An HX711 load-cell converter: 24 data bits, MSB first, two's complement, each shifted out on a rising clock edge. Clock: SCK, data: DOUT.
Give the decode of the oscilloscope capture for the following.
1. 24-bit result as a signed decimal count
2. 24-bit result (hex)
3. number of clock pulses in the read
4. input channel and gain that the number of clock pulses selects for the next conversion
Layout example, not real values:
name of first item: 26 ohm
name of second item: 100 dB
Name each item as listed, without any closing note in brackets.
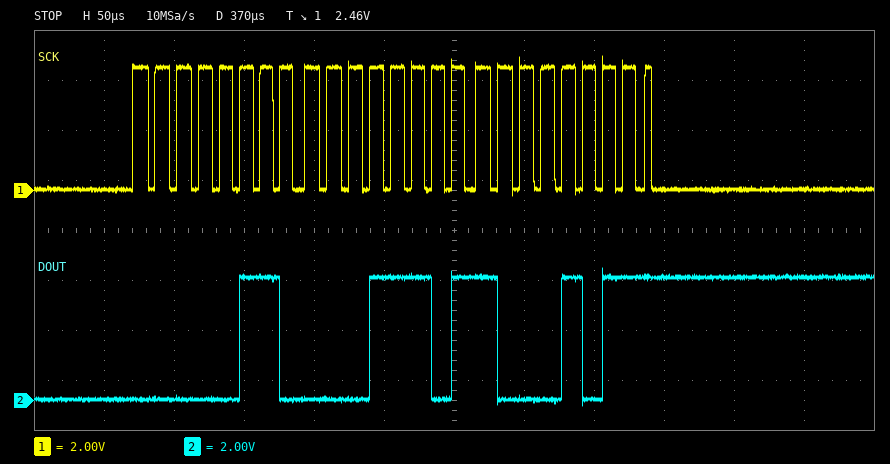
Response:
24-bit result as a signed decimal count: 400779
24-bit result: 0x061D8B
number of clock pulses in the read: 25
input channel and gain that the number of clock pulses selects for the next conversion: channel A, gain 128
